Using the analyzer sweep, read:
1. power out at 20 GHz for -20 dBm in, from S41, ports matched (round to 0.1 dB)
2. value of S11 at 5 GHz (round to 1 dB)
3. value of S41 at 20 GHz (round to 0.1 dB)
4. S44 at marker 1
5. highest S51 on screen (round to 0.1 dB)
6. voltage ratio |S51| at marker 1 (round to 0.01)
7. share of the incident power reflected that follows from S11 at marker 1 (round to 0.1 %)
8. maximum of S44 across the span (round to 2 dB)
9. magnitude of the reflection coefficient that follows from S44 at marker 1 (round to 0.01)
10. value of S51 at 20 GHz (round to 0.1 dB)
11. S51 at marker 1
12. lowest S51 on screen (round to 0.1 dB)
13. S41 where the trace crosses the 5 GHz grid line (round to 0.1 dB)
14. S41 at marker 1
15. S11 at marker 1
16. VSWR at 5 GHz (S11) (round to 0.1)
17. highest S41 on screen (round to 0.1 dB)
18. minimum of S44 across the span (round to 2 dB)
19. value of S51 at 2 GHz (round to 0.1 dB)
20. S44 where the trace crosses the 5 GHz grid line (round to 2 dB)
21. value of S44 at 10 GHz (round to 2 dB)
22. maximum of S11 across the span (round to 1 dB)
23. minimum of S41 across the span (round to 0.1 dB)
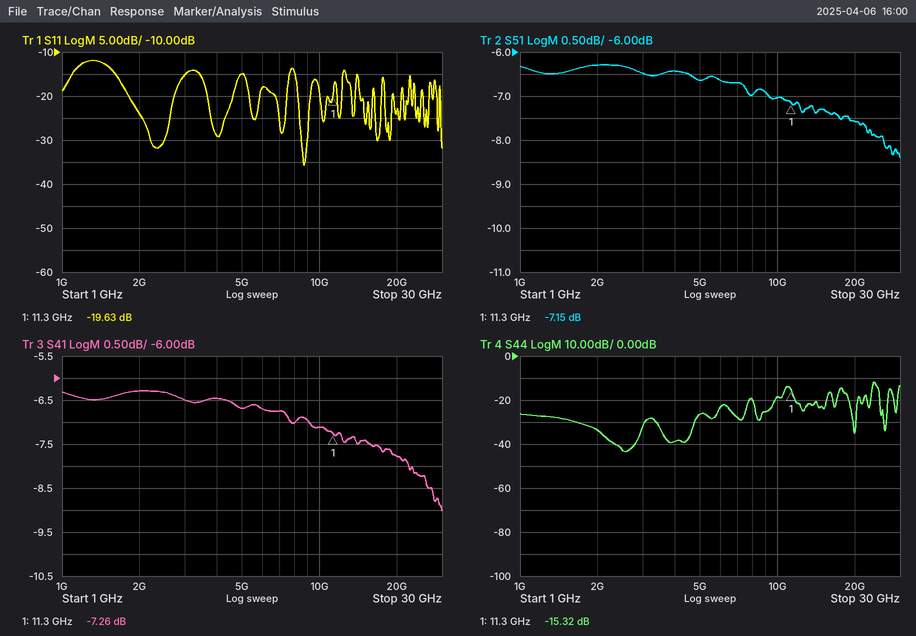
-27.8 dBm
-15 dB
-7.8 dB
-15.32 dB
-6.3 dB
0.44
1.1 %
-12 dB
0.17
-7.6 dB
-7.15 dB
-8.4 dB
-6.7 dB
-7.26 dB
-19.63 dB
1.4
-6.3 dB
-44 dB
-6.3 dB
-26 dB
-18 dB
-12 dB
-9.0 dB
